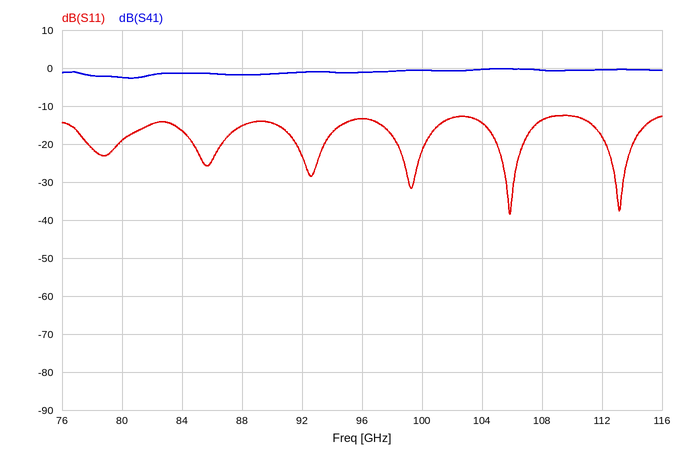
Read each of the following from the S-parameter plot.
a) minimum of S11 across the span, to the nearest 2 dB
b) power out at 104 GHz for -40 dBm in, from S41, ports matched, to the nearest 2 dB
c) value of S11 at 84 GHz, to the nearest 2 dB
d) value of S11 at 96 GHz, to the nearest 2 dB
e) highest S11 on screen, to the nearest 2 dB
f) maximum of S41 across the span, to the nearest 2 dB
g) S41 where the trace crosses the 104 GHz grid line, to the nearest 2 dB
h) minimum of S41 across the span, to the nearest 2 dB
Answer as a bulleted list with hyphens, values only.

- -38 dB
- -40 dBm
- -16 dB
- -14 dB
- -12 dB
- 0 dB
- 0 dB
- -2 dB
